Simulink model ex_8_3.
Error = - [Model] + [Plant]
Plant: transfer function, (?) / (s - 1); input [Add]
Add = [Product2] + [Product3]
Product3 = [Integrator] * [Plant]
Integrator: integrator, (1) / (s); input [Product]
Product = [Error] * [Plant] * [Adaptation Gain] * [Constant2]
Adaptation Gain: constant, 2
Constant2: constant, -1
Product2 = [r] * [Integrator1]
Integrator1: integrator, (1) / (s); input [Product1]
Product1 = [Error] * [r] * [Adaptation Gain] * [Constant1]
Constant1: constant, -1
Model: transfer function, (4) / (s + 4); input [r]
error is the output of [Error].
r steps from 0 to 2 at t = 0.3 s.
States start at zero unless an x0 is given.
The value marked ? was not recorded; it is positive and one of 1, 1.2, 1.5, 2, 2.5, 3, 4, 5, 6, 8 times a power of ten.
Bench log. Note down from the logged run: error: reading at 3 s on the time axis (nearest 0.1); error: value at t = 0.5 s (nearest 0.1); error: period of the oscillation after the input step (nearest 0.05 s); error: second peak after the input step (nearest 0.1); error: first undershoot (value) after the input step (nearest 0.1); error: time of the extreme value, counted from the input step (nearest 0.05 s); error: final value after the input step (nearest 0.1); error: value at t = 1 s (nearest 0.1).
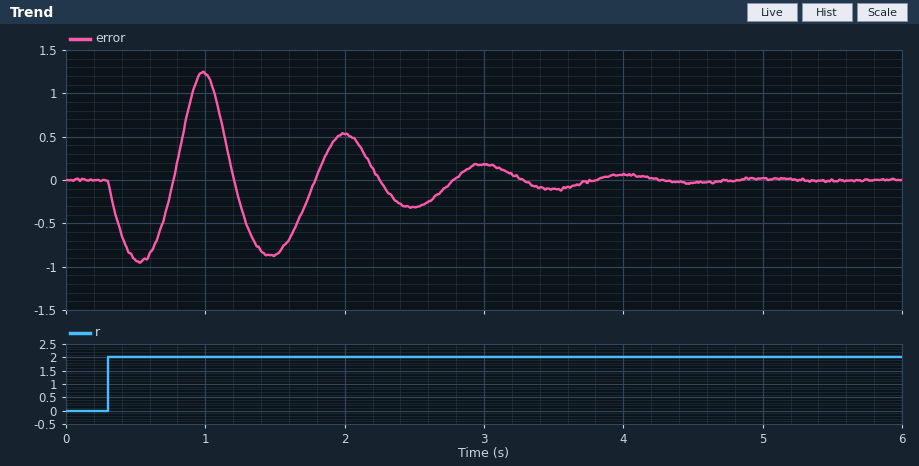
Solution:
0.2
-0.9
1.00 s
0.5
-0.9
0.70 s
0.0
1.2
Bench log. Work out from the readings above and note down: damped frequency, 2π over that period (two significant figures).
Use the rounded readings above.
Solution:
6.3 rad/s
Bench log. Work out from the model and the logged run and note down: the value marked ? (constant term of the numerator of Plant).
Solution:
2.5
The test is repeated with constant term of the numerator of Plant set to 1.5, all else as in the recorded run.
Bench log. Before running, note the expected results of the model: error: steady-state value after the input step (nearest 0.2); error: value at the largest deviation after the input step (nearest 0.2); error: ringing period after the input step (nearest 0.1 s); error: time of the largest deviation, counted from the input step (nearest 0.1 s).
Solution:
0.0
1.4
1.3 s
0.8 s
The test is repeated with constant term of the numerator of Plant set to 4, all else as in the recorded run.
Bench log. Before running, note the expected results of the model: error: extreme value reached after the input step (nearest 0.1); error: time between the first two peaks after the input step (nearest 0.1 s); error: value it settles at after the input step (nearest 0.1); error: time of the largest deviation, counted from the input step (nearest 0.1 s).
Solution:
1.1
0.8 s
0.0
0.6 s
